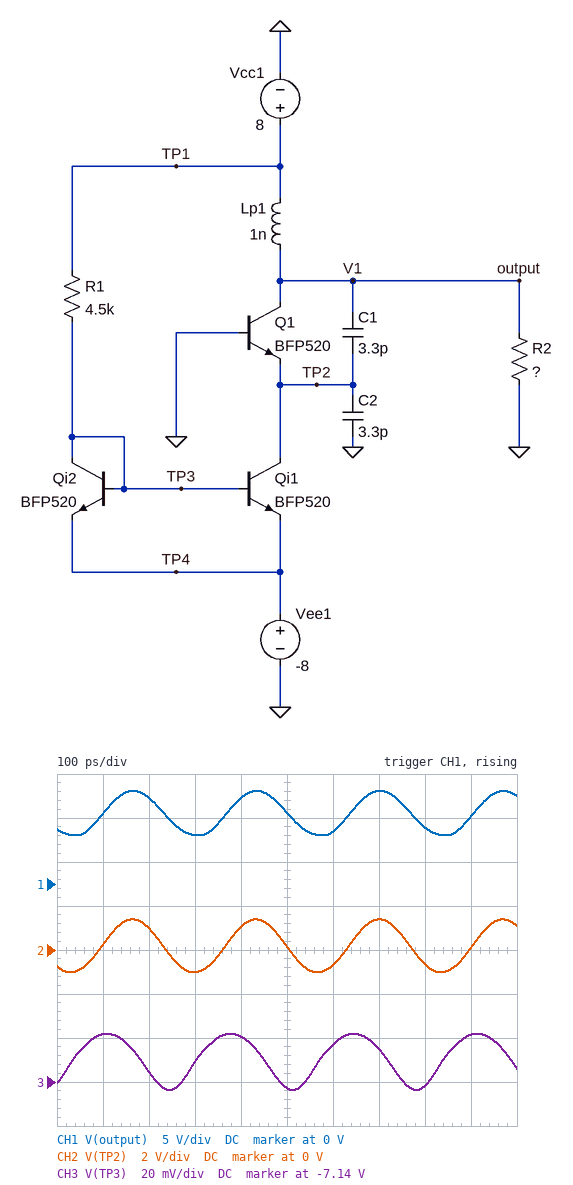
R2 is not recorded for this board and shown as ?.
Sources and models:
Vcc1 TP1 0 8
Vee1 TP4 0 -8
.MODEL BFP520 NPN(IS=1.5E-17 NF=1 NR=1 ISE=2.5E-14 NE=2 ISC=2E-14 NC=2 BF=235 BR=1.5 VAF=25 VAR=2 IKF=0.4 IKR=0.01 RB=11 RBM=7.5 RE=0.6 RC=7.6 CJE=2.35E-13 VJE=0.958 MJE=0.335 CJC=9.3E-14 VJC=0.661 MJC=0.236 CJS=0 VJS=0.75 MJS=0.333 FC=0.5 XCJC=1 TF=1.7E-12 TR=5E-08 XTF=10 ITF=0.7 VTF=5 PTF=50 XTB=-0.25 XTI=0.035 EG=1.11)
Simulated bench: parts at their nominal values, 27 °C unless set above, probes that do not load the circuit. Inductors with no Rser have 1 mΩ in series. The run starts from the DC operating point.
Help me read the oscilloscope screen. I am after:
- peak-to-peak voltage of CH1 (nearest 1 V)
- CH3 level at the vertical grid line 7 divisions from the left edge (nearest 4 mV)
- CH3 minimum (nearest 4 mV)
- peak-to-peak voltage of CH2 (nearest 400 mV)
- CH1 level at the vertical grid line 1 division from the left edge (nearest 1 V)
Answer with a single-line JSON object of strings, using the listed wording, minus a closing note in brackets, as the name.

{"peak-to-peak voltage of CH1": "5 V", "CH3 level at the vertical grid line 7 divisions from the left edge": "-7.124 V", "CH3 minimum": "-7.144 V", "peak-to-peak voltage of CH2": "2.4 V", "CH1 level at the vertical grid line 1 division from the left edge": "8 V"}
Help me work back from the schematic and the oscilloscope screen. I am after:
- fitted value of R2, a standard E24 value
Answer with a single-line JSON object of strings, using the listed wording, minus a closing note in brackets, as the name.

{"fitted value of R2, a standard E24 value": "620 Ω"}
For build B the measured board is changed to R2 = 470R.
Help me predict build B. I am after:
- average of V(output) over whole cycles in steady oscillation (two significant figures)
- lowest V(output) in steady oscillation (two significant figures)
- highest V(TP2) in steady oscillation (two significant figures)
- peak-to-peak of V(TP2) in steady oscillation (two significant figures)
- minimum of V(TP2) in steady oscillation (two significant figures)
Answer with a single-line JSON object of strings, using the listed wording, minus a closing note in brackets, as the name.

{"average of V(output) over whole cycles in steady oscillation": "8.0 V", "lowest V(output) in steady oscillation": "6.1 V", "highest V(TP2) in steady oscillation": "820 mV", "peak-to-peak of V(TP2) in steady oscillation": "1.8 V", "minimum of V(TP2) in steady oscillation": "-990 mV"}
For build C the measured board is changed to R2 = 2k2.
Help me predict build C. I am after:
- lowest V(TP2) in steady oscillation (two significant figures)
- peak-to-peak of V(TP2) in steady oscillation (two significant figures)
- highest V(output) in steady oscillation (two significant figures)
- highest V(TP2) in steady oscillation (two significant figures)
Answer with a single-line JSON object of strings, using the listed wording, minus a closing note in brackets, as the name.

{"lowest V(TP2) in steady oscillation": "-1.4 V", "peak-to-peak of V(TP2) in steady oscillation": "8.6 V", "highest V(output) in steady oscillation": "17 V", "highest V(TP2) in steady oscillation": "7.2 V"}
